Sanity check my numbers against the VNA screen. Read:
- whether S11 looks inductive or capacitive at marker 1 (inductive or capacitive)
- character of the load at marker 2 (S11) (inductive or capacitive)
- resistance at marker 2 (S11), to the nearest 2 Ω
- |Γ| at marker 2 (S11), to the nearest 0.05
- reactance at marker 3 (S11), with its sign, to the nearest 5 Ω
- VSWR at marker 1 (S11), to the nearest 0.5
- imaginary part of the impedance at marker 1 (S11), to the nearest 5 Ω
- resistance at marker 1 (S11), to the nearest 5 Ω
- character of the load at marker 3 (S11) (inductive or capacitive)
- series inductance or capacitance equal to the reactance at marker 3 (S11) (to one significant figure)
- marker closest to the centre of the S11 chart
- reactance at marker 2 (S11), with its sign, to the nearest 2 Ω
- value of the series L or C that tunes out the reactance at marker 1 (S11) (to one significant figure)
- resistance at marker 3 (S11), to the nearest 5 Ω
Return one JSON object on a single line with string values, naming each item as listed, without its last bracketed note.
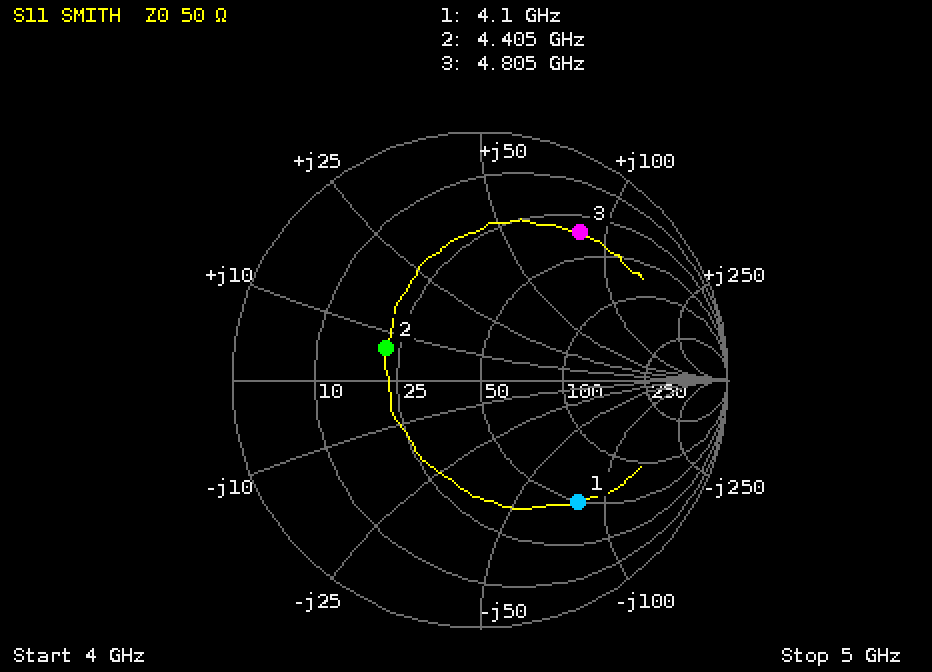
{"whether S11 looks inductive or capacitive at marker 1": "capacitive", "character of the load at marker 2 (S11)": "inductive", "resistance at marker 2 (S11), to the nearest 2 Ω": "22 Ω", "|Γ| at marker 2 (S11), to the nearest 0.05": "0.40", "reactance at marker 3 (S11), with its sign, to the nearest 5 Ω": "+85 Ω", "VSWR at marker 1 (S11), to the nearest 0.5": "4.5", "imaginary part of the impedance at marker 1 (S11), to the nearest 5 Ω": "-80 Ω", "resistance at marker 1 (S11), to the nearest 5 Ω": "50 Ω", "character of the load at marker 3 (S11)": "inductive", "series inductance or capacitance equal to the reactance at marker 3 (S11)": "3 nH", "marker closest to the centre of the S11 chart": "marker 2", "reactance at marker 2 (S11), with its sign, to the nearest 2 Ω": "+6 Ω", "value of the series L or C that tunes out the reactance at marker 1 (S11)": "3 nH", "resistance at marker 3 (S11), to the nearest 5 Ω": "35 Ω"}
